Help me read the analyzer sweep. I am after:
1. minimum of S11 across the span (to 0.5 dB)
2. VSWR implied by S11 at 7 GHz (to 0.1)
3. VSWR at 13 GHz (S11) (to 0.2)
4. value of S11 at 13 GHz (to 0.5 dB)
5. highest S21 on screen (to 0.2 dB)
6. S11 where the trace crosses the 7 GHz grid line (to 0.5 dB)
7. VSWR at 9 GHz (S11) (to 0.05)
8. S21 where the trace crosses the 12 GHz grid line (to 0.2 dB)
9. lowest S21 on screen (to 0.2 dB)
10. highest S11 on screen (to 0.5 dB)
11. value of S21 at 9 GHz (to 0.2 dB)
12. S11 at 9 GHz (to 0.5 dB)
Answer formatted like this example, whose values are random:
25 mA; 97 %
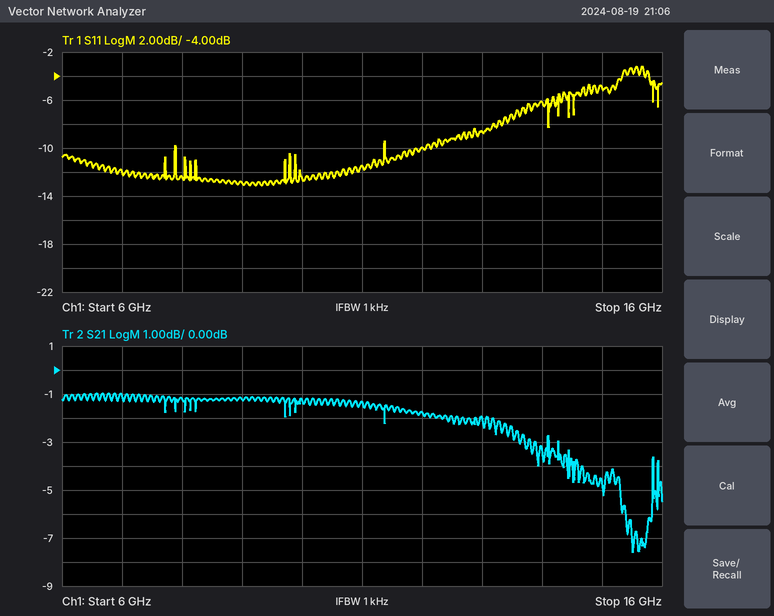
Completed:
-13.0 dB; 1.7; 2.2; -8.5 dB; -1.0 dB; -12.0 dB; 1.60; -1.8 dB; -7.6 dB; -3.0 dB; -1.2 dB; -13.0 dB
